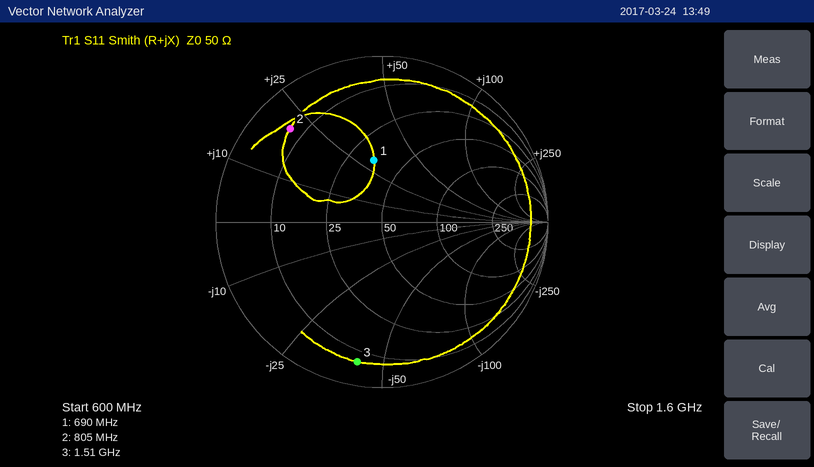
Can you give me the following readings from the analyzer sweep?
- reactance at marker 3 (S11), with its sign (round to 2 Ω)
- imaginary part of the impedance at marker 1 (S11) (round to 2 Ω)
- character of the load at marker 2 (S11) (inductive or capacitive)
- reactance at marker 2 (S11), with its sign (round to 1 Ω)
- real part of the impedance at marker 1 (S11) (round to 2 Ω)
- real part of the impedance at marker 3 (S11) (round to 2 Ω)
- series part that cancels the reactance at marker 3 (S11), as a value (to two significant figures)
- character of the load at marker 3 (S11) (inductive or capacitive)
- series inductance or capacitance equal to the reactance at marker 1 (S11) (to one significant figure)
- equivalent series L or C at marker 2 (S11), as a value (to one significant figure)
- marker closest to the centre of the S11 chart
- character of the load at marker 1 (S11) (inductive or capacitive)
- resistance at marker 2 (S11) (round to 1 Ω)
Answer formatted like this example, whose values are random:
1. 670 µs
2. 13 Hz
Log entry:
1. -42 Ω
2. +30 Ω
3. inductive
4. +21 Ω
5. 34 Ω
6. 6 Ω
7. 4.4 nH
8. capacitive
9. 7 nH
10. 4 nH
11. marker 1
12. inductive
13. 7 Ω
